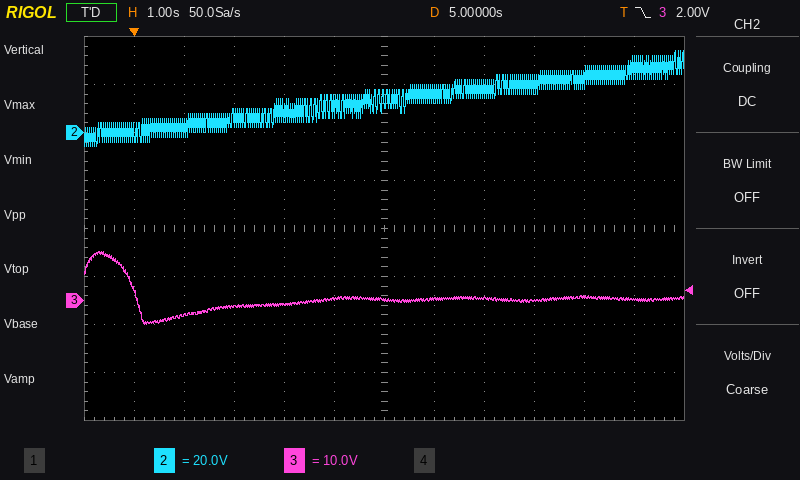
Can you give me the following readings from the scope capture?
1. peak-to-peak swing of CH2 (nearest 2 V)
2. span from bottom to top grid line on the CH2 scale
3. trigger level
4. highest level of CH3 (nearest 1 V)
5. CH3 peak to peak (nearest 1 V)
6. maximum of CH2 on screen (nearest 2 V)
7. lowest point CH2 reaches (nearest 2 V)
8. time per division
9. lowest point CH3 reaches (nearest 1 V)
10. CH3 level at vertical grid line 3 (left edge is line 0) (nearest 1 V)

40 V
160 V
2.00 V
10 V
15 V
34 V
-6 V
1 s
-5 V
-1 V
